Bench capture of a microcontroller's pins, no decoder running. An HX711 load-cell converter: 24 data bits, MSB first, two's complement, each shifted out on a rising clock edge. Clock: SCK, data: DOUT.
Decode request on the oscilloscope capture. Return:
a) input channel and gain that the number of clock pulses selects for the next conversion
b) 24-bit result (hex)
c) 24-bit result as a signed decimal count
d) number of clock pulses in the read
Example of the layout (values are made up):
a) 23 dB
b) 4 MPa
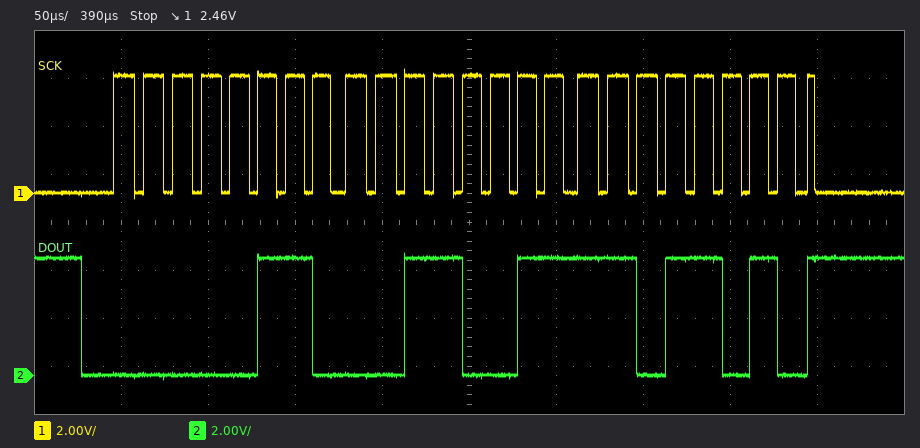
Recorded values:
a) channel A, gain 128
b) 0x0633DA
c) 406490
d) 25
